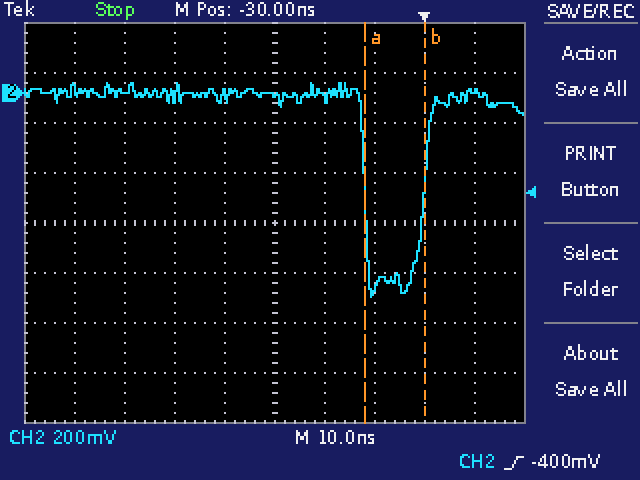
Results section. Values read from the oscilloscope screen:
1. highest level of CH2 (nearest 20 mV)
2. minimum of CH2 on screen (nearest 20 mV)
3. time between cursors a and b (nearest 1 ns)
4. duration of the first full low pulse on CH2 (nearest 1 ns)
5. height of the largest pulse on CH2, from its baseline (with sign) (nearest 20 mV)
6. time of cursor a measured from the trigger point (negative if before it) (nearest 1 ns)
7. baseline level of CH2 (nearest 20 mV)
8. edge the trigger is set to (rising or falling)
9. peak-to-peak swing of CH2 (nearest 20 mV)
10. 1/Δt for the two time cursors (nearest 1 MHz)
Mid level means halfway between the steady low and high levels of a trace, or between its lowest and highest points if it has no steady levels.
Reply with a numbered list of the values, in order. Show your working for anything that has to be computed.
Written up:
1. 40 mV
2. -820 mV
3. 12 ns
4. 12 ns
5. -820 mV − (0 mV) = -820 mV
6. -12 ns
7. 0 mV
8. rising
9. 40 mV − (-820 mV) = 860 mV
10. 1 / 12 ns ≈ 83 MHz
